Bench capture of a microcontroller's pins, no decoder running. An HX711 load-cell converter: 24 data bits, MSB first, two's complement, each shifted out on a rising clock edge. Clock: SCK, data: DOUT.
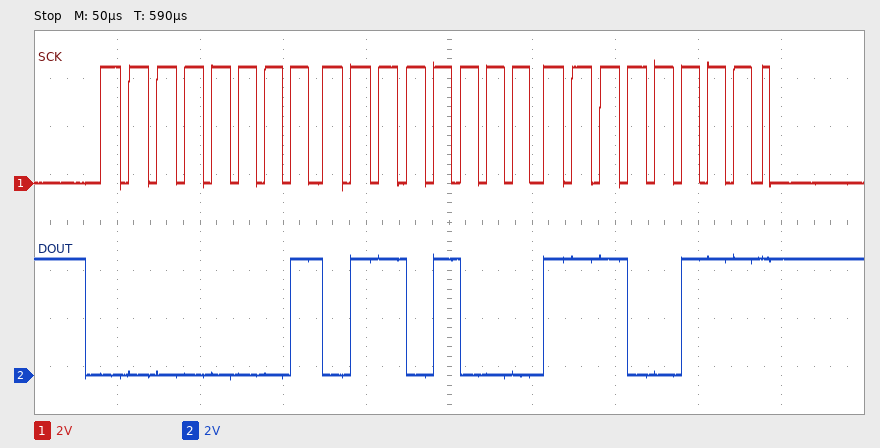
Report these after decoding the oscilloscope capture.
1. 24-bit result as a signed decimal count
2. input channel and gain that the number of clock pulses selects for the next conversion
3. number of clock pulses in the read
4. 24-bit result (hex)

92391
channel A, gain 128
25
0x0168E7
